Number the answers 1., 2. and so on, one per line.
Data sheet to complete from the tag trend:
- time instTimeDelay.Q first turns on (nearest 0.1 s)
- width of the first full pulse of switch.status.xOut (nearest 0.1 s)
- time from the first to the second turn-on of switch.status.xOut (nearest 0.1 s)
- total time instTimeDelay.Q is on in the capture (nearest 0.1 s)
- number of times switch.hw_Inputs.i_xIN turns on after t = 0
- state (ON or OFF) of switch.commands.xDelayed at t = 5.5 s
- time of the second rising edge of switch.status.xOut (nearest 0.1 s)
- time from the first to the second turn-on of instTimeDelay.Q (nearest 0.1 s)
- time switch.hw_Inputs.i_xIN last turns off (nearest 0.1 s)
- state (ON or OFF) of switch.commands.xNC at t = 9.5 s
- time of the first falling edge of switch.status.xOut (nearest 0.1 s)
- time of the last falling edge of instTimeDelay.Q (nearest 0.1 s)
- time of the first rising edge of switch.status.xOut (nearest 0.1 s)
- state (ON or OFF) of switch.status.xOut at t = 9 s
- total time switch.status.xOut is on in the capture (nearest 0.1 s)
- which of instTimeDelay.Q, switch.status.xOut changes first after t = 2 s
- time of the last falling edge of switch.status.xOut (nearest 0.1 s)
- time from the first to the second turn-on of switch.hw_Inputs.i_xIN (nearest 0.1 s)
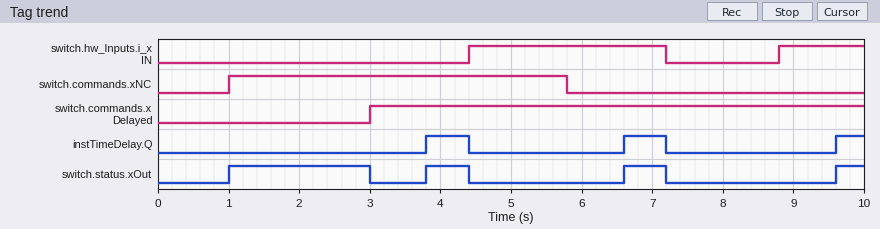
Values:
1. 3.8 s
2. 2.0 s
3. 2.8 s
4. 1.6 s
5. 2
6. ON
7. 3.8 s
8. 2.8 s
9. 7.2 s
10. OFF
11. 3.0 s
12. 7.2 s
13. 1.0 s
14. OFF
15. 3.6 s
16. switch.status.xOut
17. 7.2 s
18. 4.4 s
